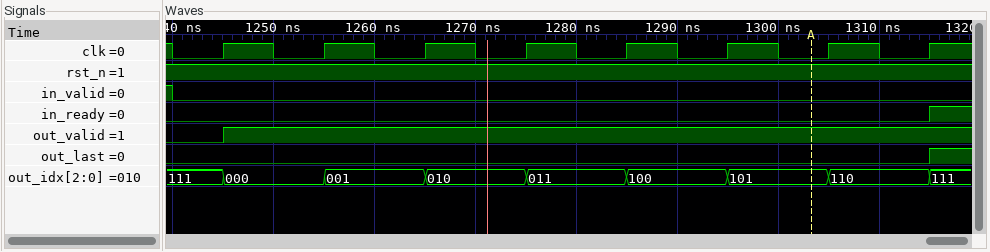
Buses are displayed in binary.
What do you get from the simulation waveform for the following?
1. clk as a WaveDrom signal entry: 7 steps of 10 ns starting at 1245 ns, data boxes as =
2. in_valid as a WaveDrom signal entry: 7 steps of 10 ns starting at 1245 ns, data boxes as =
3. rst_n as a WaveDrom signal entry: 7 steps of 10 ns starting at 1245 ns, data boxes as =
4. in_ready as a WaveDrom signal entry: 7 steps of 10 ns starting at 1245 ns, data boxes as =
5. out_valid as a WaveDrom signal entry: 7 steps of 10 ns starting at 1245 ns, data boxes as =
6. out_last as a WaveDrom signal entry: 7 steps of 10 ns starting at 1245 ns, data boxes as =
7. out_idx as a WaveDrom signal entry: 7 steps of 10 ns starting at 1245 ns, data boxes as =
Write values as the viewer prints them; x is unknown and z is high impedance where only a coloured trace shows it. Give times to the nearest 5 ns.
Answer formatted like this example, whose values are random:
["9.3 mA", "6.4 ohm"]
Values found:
["{name: 'clk', wave: 'p......'}", "{name: 'in_valid', wave: '0......'}", "{name: 'rst_n', wave: '1......'}", "{name: 'in_ready', wave: '0......'}", "{name: 'out_valid', wave: '1......'}", "{name: 'out_last', wave: '0......'}", "{name: 'out_idx', wave: '=======', data: '000 001 010 011 100 101 110'}"]
